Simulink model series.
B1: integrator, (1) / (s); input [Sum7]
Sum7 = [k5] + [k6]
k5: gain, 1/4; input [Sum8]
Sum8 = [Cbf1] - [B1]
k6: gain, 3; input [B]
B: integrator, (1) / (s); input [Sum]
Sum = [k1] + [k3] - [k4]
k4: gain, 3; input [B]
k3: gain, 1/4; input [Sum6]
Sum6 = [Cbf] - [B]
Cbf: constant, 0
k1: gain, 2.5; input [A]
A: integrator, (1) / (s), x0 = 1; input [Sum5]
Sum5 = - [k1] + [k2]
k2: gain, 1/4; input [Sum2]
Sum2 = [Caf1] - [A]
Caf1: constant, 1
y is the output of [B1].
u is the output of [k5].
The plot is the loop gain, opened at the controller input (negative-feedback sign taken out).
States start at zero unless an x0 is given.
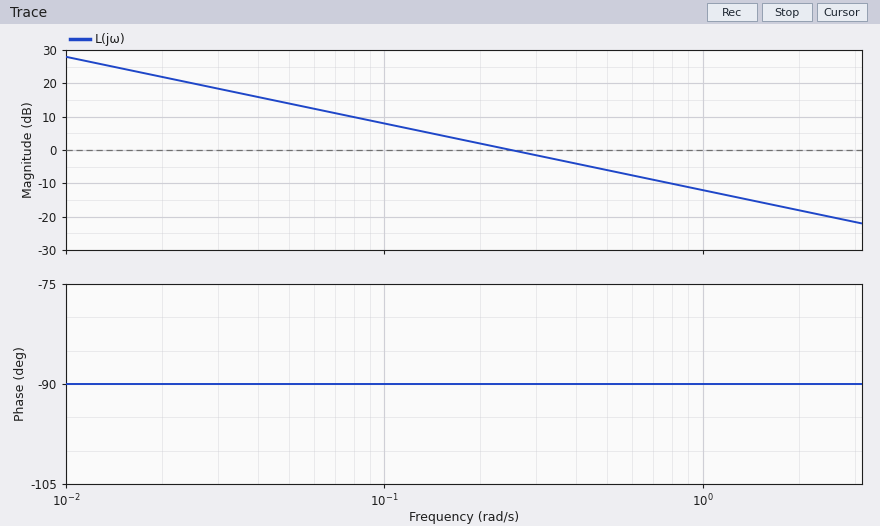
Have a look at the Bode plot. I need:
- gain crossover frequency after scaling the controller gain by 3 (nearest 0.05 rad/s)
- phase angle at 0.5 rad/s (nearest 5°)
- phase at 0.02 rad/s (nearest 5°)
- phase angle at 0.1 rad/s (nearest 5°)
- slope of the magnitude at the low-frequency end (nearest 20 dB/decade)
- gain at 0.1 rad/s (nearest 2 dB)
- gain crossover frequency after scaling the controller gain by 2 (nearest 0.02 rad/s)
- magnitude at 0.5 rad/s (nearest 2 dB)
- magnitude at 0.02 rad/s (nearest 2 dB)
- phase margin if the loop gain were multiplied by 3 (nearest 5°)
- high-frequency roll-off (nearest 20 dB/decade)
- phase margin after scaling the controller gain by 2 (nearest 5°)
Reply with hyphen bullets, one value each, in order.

- 0.75 rad/s
- -90°
- -90°
- -90°
- -20 dB/decade
- 8 dB
- 0.50 rad/s
- -6 dB
- 22 dB
- 90°
- -20 dB/decade
- 90°
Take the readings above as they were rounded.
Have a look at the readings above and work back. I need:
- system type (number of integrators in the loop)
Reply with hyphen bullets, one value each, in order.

- 1
